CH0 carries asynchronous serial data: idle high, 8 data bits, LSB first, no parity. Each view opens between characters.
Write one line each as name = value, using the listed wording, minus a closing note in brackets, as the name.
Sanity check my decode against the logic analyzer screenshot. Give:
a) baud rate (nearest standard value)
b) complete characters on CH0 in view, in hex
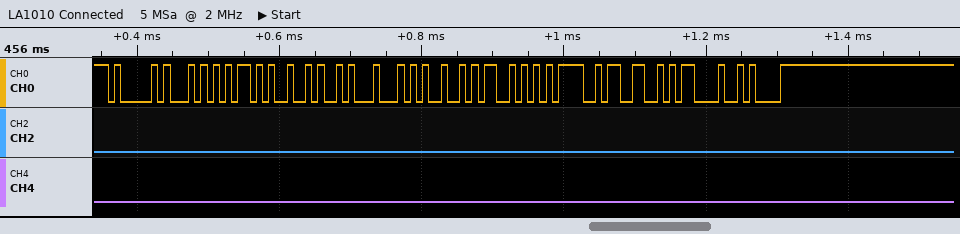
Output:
baud rate = 115200 baud
complete characters on CH0 in view, in hex = 41, 54, 2B, 4A, 44, 49, 53, 3D, 33, 0D, 0A
